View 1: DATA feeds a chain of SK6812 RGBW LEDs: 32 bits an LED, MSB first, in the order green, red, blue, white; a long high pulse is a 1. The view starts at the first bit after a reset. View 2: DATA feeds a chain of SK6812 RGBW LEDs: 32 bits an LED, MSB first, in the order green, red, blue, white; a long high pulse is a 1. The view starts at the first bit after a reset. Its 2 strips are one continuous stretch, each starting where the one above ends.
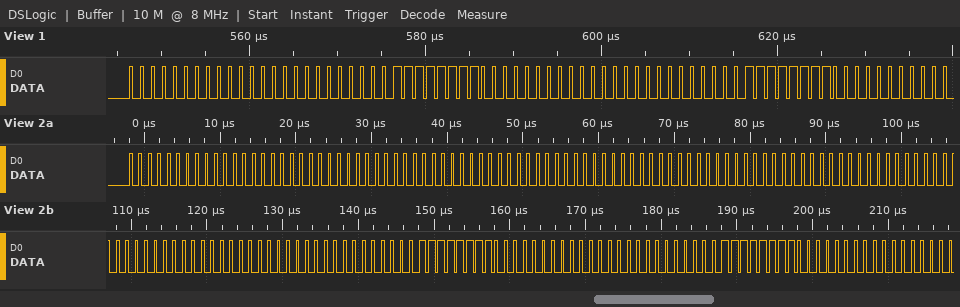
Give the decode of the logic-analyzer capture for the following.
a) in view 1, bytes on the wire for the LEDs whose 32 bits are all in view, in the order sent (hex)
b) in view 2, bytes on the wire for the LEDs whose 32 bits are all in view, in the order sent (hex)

00 00 00 FF 00 00 00 FF
00 00 00 00 00 00 00 00 00 00 00 00 00 00 00 FF 00 00 00 FF
